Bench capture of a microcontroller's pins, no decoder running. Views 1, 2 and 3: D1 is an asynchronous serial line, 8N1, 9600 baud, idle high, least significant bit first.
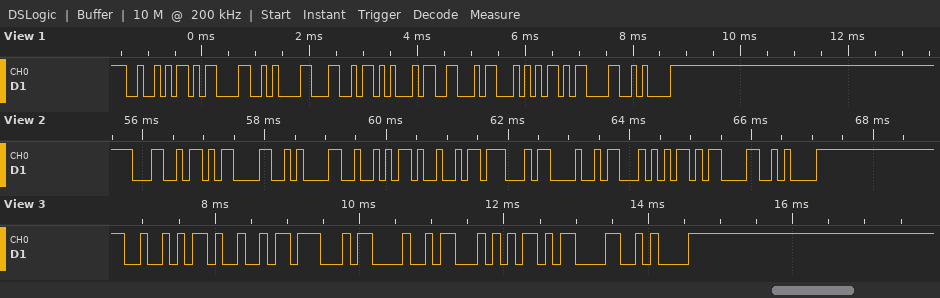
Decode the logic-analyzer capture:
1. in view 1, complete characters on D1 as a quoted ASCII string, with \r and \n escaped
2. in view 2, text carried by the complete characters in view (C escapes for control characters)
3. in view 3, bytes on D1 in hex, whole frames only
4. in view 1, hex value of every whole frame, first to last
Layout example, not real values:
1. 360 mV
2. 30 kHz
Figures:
1. "R\r\nLEFT\r\n"
2. "L\r\nRIGHT\r\n"
3. 52 49 47 48 54 0D 0A
4. 52 0D 0A 4C 45 46 54 0D 0A
